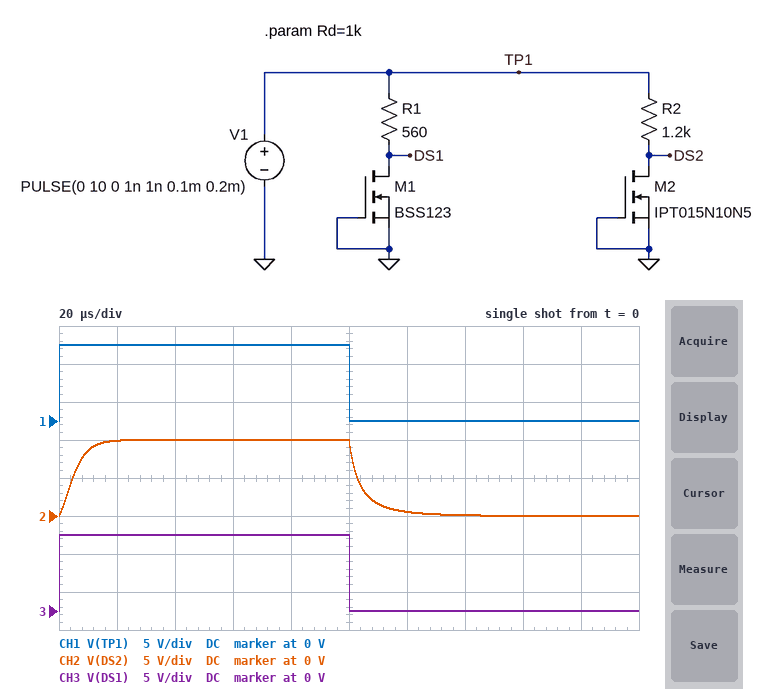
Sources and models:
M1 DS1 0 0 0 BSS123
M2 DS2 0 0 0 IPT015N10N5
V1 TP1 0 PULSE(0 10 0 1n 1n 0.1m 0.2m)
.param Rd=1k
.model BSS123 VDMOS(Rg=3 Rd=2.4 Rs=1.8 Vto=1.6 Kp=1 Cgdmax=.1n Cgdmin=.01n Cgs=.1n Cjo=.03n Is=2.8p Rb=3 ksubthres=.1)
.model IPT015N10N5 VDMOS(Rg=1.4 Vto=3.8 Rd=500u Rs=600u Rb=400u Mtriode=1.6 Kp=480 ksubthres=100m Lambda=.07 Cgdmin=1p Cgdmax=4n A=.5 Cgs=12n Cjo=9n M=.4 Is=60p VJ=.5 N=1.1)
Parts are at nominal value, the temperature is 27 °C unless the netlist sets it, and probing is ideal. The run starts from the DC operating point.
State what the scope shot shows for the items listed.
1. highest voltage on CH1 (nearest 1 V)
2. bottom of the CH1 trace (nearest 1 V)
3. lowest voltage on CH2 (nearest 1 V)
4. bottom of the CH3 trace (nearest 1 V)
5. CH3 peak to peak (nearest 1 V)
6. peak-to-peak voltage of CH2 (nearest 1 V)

10 V
0 V
0 V
0 V
10 V
10 V
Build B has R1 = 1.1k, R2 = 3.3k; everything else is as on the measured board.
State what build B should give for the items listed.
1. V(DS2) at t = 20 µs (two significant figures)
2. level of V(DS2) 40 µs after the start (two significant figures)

7.2 V
9.6 V
